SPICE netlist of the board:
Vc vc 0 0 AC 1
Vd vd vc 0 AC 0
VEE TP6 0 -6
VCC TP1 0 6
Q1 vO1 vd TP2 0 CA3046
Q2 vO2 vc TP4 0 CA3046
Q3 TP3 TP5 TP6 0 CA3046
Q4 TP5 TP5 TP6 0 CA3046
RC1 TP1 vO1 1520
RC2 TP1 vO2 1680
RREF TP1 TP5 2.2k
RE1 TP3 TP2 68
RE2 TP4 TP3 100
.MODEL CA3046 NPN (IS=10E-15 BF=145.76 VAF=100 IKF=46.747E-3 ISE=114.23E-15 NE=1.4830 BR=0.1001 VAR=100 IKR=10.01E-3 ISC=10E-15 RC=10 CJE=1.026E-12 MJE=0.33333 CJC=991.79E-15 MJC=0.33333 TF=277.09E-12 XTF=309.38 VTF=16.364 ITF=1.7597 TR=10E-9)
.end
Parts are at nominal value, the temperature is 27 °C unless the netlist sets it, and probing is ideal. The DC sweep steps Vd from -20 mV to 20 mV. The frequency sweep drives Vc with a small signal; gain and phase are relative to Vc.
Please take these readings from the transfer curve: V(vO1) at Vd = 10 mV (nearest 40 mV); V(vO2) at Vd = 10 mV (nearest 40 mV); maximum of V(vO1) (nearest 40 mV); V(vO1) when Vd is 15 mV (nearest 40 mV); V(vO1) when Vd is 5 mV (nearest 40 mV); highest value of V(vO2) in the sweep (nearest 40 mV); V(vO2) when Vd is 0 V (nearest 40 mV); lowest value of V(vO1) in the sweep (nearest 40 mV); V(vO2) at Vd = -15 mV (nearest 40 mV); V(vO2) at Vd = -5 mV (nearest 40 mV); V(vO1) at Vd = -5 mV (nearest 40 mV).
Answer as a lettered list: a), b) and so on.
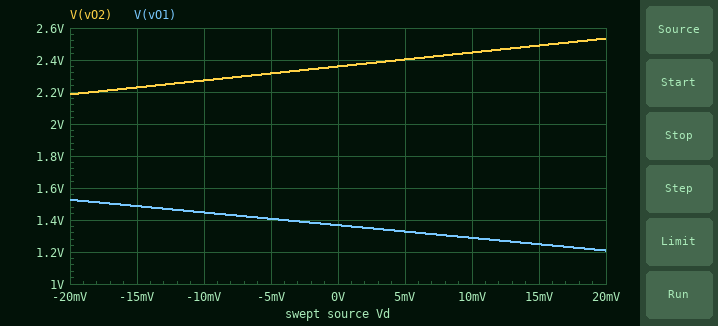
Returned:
a) 1.28 V
b) 2.44 V
c) 1.52 V
d) 1.24 V
e) 1.32 V
f) 2.52 V
g) 2.36 V
h) 1.20 V
i) 2.24 V
j) 2.32 V
k) 1.40 V
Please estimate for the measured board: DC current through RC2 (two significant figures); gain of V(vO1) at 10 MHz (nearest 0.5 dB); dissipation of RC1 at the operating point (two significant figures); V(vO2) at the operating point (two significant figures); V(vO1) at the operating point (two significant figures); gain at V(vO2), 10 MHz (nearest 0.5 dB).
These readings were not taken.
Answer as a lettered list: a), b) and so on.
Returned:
a) 2.2 mA
b) -26.5 dB
c) 14 mW
d) 2.4 V
e) 1.4 V
f) -27.5 dB
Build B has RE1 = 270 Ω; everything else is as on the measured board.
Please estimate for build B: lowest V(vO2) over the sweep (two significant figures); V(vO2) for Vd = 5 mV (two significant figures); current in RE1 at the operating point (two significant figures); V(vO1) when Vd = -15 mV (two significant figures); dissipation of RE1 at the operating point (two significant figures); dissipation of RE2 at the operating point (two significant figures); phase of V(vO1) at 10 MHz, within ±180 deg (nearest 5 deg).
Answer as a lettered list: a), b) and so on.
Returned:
a) -350 mV
b) -240 mV
c) 1.5 mA
d) 3.8 V
e) 600 µW
f) 1.4 mW
g) 125 deg
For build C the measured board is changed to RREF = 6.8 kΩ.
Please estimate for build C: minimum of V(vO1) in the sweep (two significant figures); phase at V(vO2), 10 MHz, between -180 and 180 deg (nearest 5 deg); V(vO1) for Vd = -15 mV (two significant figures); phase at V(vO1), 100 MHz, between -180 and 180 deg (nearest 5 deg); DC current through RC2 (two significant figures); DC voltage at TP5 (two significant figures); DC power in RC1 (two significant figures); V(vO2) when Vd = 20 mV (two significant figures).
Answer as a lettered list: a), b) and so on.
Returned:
a) 4.4 V
b) 140 deg
c) 4.6 V
d) 150 deg
e) 730 µA
f) -5.3 V
g) 1.4 mW
h) 4.9 V
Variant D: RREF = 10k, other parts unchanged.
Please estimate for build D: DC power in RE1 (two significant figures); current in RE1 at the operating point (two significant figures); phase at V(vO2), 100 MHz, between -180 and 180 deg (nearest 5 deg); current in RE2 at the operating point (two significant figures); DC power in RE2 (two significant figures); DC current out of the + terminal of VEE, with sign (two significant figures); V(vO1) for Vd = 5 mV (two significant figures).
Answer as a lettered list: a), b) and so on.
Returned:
a) 29 µW
b) 650 µA
c) 110 deg
d) 510 µA
e) 26 µW
f) -2.3 mA
g) 5.0 V
